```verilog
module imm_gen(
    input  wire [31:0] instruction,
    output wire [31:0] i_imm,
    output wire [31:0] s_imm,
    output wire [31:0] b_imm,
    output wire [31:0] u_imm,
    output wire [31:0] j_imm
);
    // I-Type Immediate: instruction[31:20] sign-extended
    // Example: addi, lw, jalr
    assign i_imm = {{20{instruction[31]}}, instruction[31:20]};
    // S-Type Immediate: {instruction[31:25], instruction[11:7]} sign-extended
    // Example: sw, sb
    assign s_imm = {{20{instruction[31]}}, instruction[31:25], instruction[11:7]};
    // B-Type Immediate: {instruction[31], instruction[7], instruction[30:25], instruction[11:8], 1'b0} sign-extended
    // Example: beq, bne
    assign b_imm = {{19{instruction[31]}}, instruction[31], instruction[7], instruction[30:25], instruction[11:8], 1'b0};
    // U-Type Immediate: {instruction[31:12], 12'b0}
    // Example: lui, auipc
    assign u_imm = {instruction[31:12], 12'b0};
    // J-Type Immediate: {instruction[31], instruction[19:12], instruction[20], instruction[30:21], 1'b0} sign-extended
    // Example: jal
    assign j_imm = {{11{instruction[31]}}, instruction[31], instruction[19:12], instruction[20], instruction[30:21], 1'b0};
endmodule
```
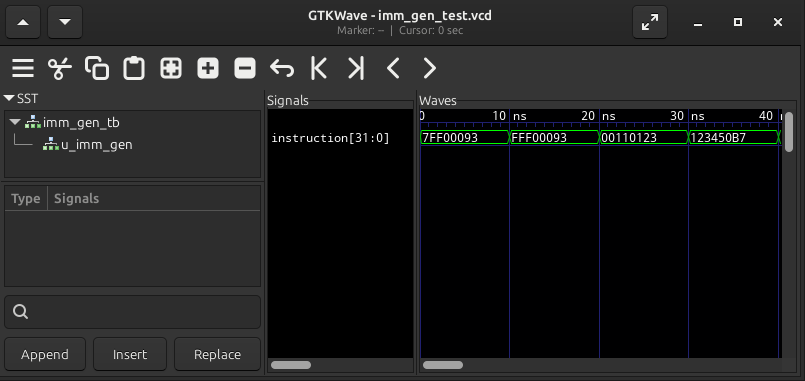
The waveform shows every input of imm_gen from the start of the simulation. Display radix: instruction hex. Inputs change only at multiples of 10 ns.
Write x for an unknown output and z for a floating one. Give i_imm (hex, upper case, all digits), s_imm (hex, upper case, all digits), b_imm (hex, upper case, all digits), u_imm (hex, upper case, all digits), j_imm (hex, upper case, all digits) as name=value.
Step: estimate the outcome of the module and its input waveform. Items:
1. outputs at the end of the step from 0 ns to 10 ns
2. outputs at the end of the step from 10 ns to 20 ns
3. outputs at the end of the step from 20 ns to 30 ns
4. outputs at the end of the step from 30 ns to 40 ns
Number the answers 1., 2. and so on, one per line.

1. i_imm=000007FF, s_imm=000007E1, b_imm=00000FE0, u_imm=7FF00000, j_imm=00000FFE
2. i_imm=FFFFFFFF, s_imm=FFFFFFE1, b_imm=FFFFFFE0, u_imm=FFF00000, j_imm=FFF00FFE
3. i_imm=00000001, s_imm=00000002, b_imm=00000002, u_imm=00110000, j_imm=00010800
4. i_imm=00000123, s_imm=00000121, b_imm=00000920, u_imm=12345000, j_imm=00045922
